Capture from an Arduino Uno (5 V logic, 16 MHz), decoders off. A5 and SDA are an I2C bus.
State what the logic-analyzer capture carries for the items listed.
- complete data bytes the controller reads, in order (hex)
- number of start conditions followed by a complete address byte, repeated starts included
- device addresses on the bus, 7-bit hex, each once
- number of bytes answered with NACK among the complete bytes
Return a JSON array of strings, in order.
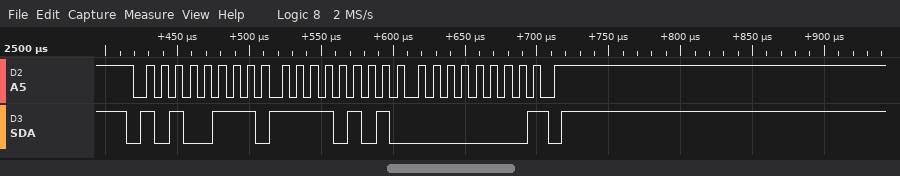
["F5 00", "1", "0x53", "1"]
